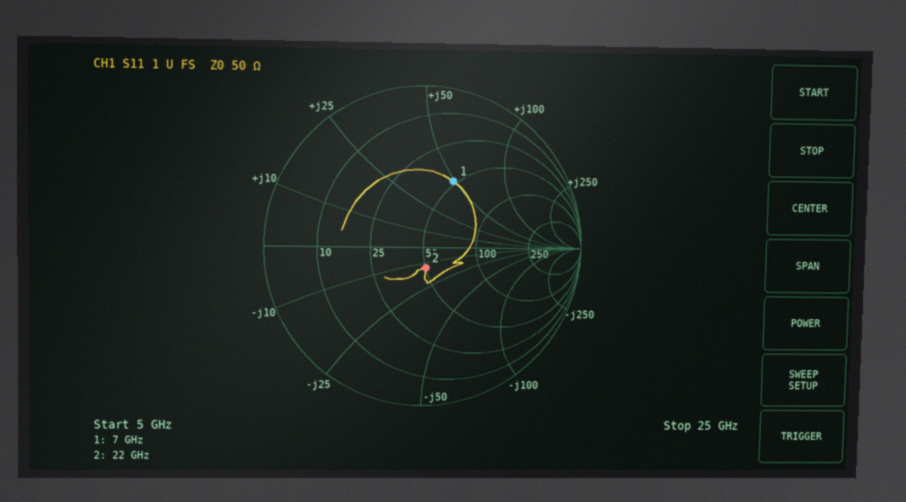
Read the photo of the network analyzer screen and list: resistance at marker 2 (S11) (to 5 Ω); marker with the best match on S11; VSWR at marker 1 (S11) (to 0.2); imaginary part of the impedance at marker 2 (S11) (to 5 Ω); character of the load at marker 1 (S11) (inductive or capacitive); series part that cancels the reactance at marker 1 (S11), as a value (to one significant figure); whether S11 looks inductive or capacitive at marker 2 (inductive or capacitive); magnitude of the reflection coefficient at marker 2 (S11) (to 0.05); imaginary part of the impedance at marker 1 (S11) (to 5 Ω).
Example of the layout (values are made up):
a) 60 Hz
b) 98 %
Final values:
a) 50 Ω
b) marker 2
c) 2.6
d) -15 Ω
e) inductive
f) 500 fF
g) capacitive
h) 0.15
i) +50 Ω
